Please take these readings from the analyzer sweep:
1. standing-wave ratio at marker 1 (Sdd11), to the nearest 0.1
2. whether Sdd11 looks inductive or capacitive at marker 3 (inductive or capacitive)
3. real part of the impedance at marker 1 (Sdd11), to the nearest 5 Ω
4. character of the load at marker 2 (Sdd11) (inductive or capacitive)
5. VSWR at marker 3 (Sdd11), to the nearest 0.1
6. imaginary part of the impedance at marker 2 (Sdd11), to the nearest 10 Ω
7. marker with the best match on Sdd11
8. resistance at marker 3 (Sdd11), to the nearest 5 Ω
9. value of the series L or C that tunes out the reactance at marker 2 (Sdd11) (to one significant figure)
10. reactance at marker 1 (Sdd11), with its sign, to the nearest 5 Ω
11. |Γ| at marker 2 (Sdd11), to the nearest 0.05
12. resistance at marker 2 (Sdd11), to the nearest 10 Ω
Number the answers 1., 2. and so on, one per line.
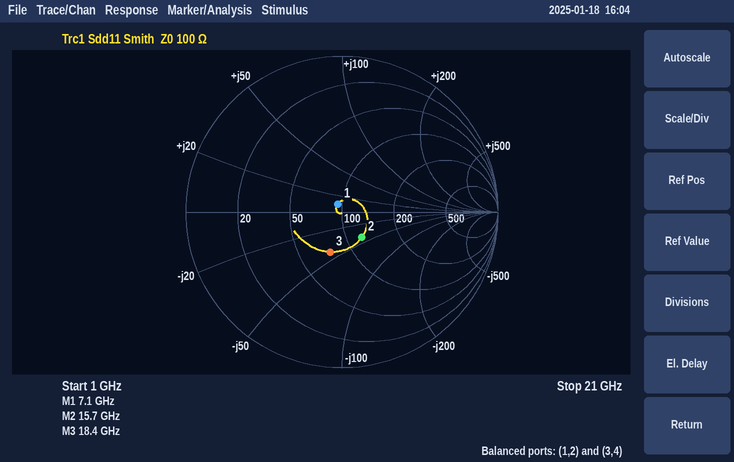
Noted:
1. 1.1
2. capacitive
3. 95 Ω
4. capacitive
5. 1.7
6. -40 Ω
7. marker 1
8. 75 Ω
9. 400 pH
10. +10 Ω
11. 0.20
12. 120 Ω
